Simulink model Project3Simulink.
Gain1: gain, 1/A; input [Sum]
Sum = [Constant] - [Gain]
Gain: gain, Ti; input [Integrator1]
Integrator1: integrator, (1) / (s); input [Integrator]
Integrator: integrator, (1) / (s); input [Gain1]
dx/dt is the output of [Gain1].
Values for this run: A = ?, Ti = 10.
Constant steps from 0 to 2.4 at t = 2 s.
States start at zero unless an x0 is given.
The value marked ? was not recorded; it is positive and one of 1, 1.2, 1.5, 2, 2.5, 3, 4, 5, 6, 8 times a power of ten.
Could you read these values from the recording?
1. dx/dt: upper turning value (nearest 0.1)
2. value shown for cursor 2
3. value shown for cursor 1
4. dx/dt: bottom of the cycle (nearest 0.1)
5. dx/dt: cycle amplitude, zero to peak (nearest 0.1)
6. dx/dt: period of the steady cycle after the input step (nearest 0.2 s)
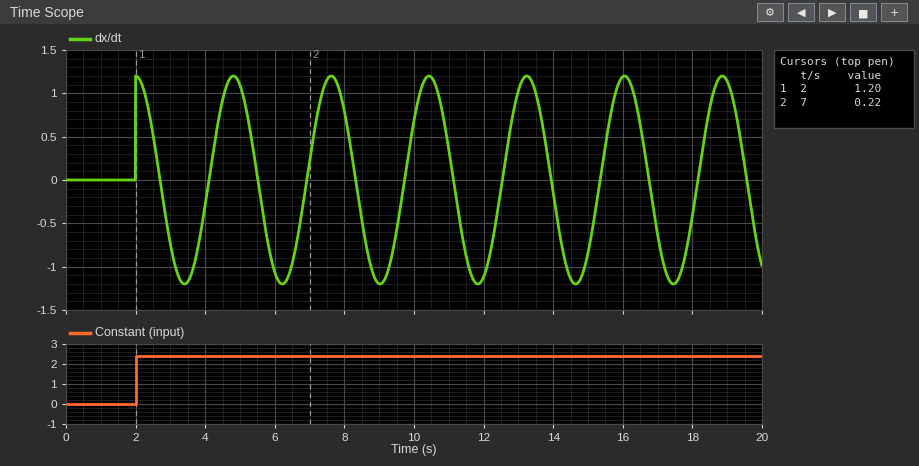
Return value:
1.2
0.22
1.20
-1.2
1.2
2.8 s
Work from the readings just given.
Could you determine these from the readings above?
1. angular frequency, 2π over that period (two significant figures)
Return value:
2.2 rad/s
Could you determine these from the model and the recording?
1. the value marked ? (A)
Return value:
2
